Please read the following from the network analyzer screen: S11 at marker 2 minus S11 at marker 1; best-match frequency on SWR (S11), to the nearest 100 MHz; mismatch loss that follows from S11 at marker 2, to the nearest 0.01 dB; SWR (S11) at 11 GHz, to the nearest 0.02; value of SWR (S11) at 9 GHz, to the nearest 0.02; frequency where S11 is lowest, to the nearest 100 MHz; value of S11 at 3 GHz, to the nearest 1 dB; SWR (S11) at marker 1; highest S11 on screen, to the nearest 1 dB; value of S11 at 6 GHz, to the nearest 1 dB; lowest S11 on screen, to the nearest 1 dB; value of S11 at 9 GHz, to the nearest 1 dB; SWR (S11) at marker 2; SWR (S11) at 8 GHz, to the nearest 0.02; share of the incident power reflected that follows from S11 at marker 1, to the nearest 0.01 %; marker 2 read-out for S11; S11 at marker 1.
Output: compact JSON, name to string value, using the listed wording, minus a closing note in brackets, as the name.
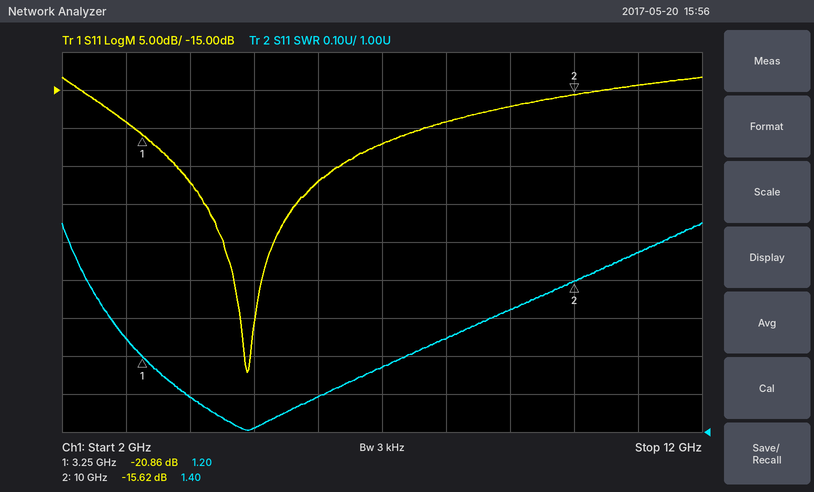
{"S11 at marker 2 minus S11 at marker 1": "5.24 dB", "best-match frequency on SWR (S11), to the nearest 100 MHz": "4.9 GHz", "mismatch loss that follows from S11 at marker 2, to the nearest 0.01 dB": "0.12 dB", "SWR (S11) at 11 GHz, to the nearest 0.02": "1.48", "value of SWR (S11) at 9 GHz, to the nearest 0.02": "1.32", "frequency where S11 is lowest, to the nearest 100 MHz": "4.9 GHz", "value of S11 at 3 GHz, to the nearest 1 dB": "-19 dB", "SWR (S11) at marker 1": "1.20", "highest S11 on screen, to the nearest 1 dB": "-13 dB", "value of S11 at 6 GHz, to the nearest 1 dB": "-27 dB", "lowest S11 on screen, to the nearest 1 dB": "-52 dB", "value of S11 at 9 GHz, to the nearest 1 dB": "-17 dB", "SWR (S11) at marker 2": "1.40", "SWR (S11) at 8 GHz, to the nearest 0.02": "1.24", "share of the incident power reflected that follows from S11 at marker 1, to the nearest 0.01 %": "0.82 %", "marker 2 read-out for S11": "-15.62 dB", "S11 at marker 1": "-20.86 dB"}
